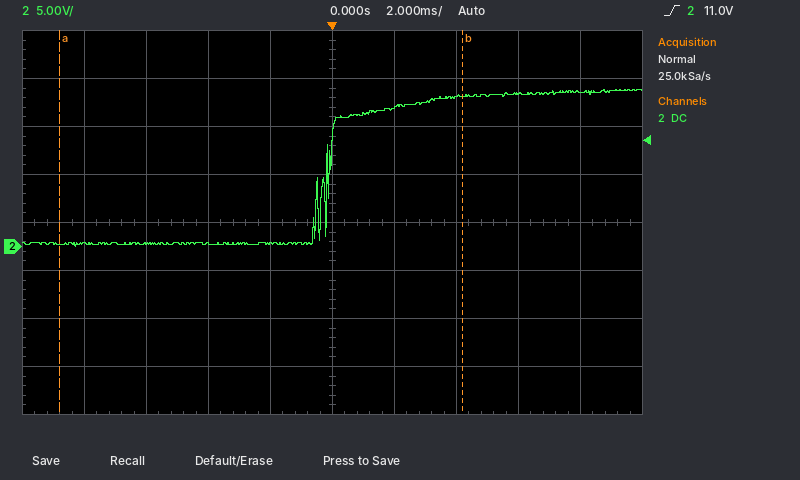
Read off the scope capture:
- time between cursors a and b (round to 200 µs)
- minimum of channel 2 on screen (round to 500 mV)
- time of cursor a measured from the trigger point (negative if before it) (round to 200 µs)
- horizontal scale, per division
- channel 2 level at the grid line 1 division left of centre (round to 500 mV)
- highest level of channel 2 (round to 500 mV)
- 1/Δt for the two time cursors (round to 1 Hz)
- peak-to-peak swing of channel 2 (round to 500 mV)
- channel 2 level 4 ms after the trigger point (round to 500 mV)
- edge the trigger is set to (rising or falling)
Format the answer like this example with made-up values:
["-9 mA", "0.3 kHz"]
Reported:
["13.0 ms", "0.0 V", "-8.8 ms", "2 ms", "500 mV", "16.5 V", "77 Hz", "16.5 V", "15.5 V", "rising"]
